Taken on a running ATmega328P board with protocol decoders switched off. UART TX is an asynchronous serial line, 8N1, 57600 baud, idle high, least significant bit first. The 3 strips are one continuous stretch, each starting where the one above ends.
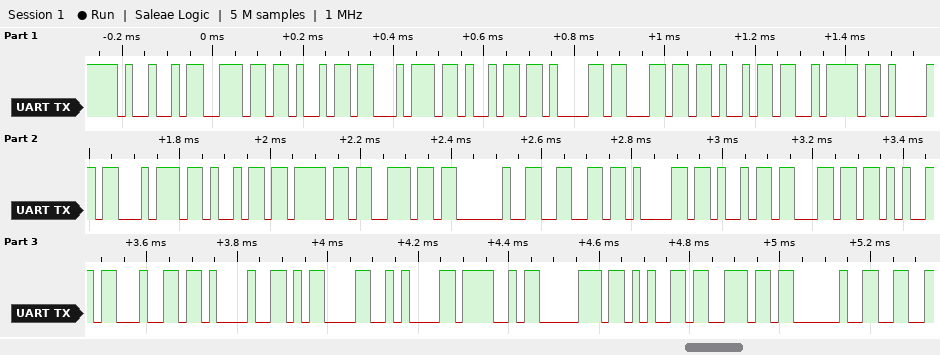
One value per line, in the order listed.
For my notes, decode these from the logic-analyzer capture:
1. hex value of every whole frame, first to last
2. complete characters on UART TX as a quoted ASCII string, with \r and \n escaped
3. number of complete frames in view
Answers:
49 6E 69 74 69 61 6C 69 7A 61 74 69 6F 6E 20 66 61 69 6C 65 64 21 0D 0A 4F 70 65 6E 20
"Initialization failed!\r\nOpen "
29
